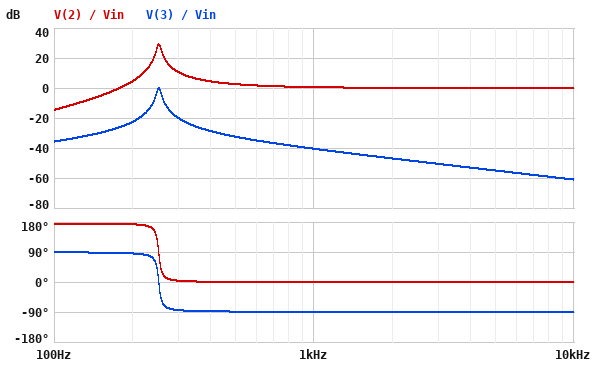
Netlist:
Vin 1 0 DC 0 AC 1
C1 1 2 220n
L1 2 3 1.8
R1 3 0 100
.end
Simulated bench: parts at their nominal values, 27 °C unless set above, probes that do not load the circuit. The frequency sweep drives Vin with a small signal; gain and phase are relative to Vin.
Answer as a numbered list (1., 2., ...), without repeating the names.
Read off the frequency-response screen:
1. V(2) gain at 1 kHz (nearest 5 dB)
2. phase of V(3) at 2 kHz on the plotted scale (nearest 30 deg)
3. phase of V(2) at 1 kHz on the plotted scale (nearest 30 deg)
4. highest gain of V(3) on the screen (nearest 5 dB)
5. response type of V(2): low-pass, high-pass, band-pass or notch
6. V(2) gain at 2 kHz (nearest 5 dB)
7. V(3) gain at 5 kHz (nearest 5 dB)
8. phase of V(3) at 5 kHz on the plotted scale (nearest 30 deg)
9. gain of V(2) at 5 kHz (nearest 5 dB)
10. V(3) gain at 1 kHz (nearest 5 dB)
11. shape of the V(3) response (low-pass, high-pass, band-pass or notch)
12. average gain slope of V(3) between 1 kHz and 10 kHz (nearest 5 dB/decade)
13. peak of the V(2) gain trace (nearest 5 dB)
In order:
1. 0 dB
2. -90 deg
3. 0 deg
4. 0 dB
5. high-pass
6. 0 dB
7. -55 dB
8. -90 deg
9. 0 dB
10. -40 dB
11. band-pass
12. -20 dB/decade
13. 30 dB
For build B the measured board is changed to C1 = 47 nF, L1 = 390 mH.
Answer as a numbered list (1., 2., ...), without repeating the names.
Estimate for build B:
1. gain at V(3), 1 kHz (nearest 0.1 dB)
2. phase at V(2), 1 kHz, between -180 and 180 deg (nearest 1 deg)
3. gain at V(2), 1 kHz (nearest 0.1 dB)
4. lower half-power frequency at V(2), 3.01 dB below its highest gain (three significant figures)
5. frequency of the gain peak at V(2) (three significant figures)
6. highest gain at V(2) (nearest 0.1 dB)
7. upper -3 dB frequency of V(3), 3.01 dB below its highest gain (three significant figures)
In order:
1. -19.5 dB
2. 172 deg
3. 8.3 dB
4. 1.16 kHz
5. 1.18 kHz
6. 29.2 dB
7. 1.20 kHz
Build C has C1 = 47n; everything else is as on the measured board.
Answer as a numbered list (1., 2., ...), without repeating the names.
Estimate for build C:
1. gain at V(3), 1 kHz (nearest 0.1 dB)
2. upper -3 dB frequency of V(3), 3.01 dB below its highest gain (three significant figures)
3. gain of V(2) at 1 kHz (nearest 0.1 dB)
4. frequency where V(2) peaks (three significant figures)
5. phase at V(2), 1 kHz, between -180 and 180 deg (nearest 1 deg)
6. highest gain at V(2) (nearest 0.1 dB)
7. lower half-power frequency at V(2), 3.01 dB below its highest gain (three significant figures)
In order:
1. -38.0 dB
2. 552 Hz
3. 3.1 dB
4. 547 Hz
5. 0 deg
6. 35.8 dB
7. 543 Hz
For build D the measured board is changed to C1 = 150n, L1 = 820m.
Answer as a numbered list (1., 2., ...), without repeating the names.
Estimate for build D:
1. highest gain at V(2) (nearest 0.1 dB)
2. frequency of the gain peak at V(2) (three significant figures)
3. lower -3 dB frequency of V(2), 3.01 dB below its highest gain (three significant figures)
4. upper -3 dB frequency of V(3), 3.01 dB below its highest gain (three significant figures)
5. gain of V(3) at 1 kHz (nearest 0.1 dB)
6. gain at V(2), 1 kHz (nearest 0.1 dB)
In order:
1. 27.4 dB
2. 454 Hz
3. 445 Hz
4. 464 Hz
5. -32.2 dB
6. 2.0 dB
